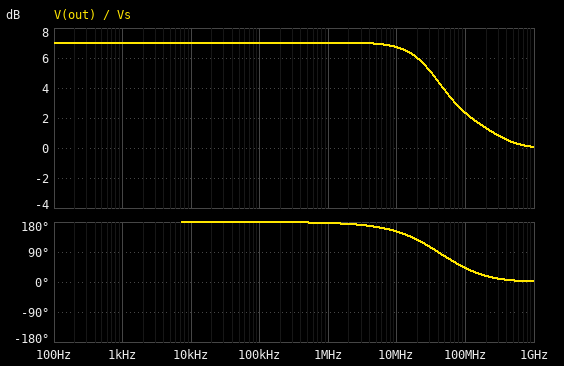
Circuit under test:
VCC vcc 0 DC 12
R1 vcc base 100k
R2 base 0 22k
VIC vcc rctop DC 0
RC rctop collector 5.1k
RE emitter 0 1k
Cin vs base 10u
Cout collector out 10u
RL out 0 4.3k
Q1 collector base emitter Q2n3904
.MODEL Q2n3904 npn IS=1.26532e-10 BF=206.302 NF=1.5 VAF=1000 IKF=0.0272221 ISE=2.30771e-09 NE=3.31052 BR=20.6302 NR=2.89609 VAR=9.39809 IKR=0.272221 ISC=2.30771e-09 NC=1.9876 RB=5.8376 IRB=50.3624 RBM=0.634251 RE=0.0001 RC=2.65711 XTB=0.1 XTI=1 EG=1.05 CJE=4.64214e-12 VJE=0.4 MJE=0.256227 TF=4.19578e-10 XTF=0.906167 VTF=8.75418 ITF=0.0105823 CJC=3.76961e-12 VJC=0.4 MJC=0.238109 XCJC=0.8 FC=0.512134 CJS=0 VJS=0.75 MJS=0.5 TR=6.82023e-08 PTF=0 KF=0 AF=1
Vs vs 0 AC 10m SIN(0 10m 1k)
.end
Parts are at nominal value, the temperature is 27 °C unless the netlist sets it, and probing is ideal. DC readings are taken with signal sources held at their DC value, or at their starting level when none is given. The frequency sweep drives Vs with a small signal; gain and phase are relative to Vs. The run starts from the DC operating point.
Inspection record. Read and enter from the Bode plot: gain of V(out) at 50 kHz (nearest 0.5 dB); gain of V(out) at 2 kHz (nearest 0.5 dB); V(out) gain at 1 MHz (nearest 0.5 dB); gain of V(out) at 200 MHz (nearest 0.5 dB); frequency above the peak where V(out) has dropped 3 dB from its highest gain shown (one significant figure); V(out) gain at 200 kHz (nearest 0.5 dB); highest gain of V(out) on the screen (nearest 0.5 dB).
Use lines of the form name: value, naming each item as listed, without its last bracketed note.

gain of V(out) at 50 kHz: 7.0 dB
gain of V(out) at 2 kHz: 7.0 dB
V(out) gain at 1 MHz: 7.0 dB
gain of V(out) at 200 MHz: 1.5 dB
frequency above the peak where V(out) has dropped 3 dB from its highest gain shown: 50 MHz
V(out) gain at 200 kHz: 7.0 dB
highest gain of V(out) on the screen: 7.0 dB
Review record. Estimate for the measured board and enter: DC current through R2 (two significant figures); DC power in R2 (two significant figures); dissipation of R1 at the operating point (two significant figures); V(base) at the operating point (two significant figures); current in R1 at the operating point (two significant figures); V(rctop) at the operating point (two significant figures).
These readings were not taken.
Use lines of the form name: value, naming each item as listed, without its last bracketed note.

DC current through R2: 89 µA
DC power in R2: 180 µW
dissipation of R1 at the operating point: 1.0 mW
V(base) at the operating point: 2.0 V
current in R1 at the operating point: 100 µA
V(rctop) at the operating point: 12 V
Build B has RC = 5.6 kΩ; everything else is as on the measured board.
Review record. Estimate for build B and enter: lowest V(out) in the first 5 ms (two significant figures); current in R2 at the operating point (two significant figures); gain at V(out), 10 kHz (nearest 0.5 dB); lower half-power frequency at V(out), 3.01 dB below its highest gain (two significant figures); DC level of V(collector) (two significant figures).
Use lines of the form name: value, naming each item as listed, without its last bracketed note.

lowest V(out) in the first 5 ms: -23 mV
current in R2 at the operating point: 89 µA
gain at V(out), 10 kHz: 7.5 dB
lower half-power frequency at V(out), 3.01 dB below its highest gain: 2.0 Hz
DC level of V(collector): 4.6 V
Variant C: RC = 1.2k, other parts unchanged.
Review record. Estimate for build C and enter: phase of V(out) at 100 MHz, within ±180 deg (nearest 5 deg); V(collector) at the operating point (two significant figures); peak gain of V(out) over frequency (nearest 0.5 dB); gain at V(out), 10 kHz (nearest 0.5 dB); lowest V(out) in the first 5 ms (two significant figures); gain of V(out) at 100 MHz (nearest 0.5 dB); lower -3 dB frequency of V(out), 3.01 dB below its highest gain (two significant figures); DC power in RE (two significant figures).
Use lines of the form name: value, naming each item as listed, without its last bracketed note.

phase of V(out) at 100 MHz, within ±180 deg: 70 deg
V(collector) at the operating point: 10 V
peak gain of V(out) over frequency: 1.0 dB
gain at V(out), 10 kHz: -1.0 dB
lowest V(out) in the first 5 ms: -9.0 mV
gain of V(out) at 100 MHz: 0.5 dB
lower -3 dB frequency of V(out), 3.01 dB below its highest gain: 5.4 Hz
DC power in RE: 1.8 mW
